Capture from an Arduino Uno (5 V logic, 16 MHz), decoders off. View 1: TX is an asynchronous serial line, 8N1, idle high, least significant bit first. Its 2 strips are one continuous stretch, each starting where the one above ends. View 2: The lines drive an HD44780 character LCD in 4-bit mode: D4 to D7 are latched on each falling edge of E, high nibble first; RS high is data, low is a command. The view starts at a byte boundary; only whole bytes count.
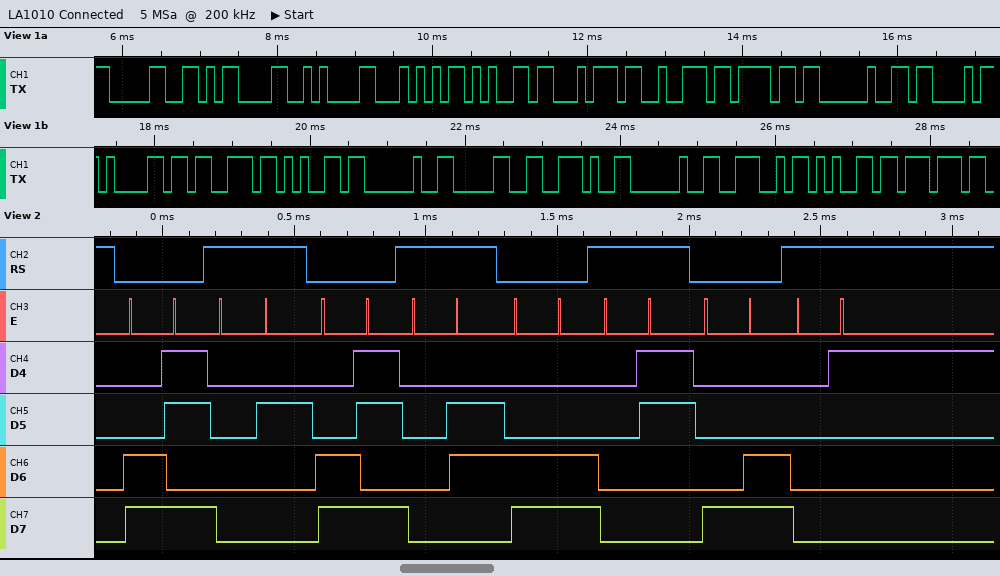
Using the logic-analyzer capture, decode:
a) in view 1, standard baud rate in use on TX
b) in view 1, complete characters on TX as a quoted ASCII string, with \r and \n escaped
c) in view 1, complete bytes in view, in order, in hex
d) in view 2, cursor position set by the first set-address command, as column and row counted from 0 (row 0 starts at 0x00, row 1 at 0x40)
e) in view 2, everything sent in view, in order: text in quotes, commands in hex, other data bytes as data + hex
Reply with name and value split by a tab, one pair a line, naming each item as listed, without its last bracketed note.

in view 1, standard baud rate in use on TX	9600 baud
in view 1, complete characters on TX as a quoted ASCII string, with \r and \n escaped	"0\r\nTetro Case 0. New"
in view 1, complete bytes in view, in order, in hex	30 0D 0A 54 65 74 72 6F 20 43 61 73 65 20 30 2E 20 4E 65 77
in view 2, cursor position set by the first set-address command, as column and row counted from 0	column 11, row 1
in view 2, everything sent in view, in order: text in quotes, commands in hex, other data bytes as data + hex	0xCB data 02 0xCB data 06 0xCC data 03 0x8C data 01
